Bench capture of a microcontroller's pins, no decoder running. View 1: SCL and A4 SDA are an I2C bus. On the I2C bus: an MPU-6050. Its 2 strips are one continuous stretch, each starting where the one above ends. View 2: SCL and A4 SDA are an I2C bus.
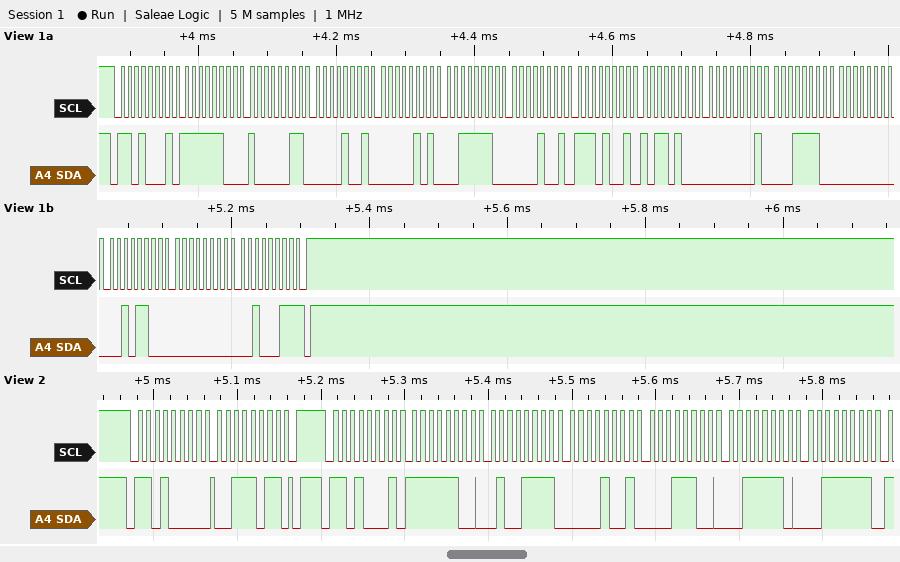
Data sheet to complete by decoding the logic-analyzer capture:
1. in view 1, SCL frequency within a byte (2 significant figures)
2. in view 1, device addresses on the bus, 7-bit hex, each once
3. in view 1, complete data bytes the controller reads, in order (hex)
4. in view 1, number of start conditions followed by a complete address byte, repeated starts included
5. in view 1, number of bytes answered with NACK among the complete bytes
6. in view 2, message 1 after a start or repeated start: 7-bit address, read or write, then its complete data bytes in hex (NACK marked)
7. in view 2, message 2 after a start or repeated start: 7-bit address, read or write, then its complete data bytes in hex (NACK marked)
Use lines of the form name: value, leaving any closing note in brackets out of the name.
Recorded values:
in view 1, SCL frequency within a byte: 100 kHz
in view 1, device addresses on the bus, 7-bit hex, each once: 0x68
in view 1, complete data bytes the controller reads, in order: FC 83 09 05 3E 09 E9 B4 01 1E 00 2C 00 23
in view 1, number of start conditions followed by a complete address byte, repeated starts included: 1
in view 1, number of bytes answered with NACK among the complete bytes: 1
in view 2, message 1 after a start or repeated start: 7-bit address, read or write, then its complete data bytes in hex: 0x68 write: 3B
in view 2, message 2 after a start or repeated start: 7-bit address, read or write, then its complete data bytes in hex: 0x68 read: FC 4F 09 1C 3E 3F
